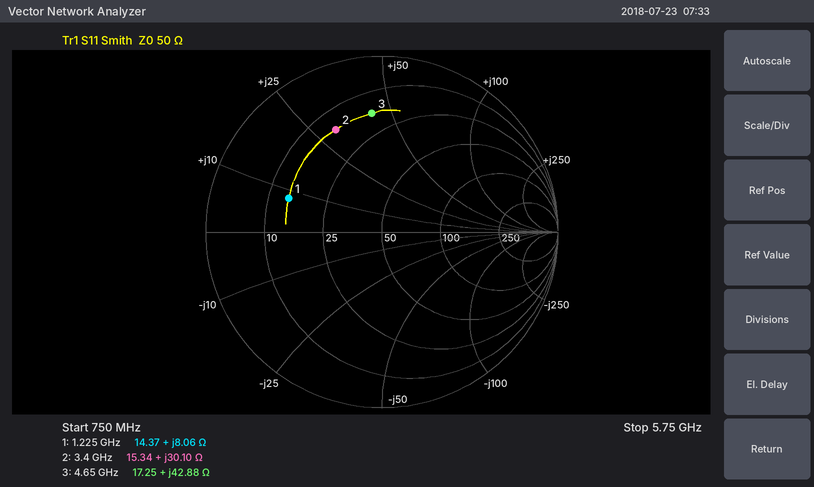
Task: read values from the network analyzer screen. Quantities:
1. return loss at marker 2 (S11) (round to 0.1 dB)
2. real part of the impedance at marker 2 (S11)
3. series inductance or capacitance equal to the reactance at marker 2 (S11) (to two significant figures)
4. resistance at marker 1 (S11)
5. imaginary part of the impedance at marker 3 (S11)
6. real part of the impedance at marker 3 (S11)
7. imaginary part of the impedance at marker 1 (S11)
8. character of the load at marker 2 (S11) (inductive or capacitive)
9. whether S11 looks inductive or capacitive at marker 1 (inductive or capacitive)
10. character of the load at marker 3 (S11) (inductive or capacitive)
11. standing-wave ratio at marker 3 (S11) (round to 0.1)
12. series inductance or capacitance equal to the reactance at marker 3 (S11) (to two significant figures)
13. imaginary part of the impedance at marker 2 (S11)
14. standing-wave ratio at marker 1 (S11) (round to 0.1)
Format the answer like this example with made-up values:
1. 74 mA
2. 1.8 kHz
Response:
1. 3.9 dB
2. 15.34 Ω
3. 1.4 nH
4. 14.37 Ω
5. +42.88 Ω
6. 17.25 Ω
7. +8.06 Ω
8. inductive
9. inductive
10. inductive
11. 5.2
12. 1.5 nH
13. +30.10 Ω
14. 3.6
